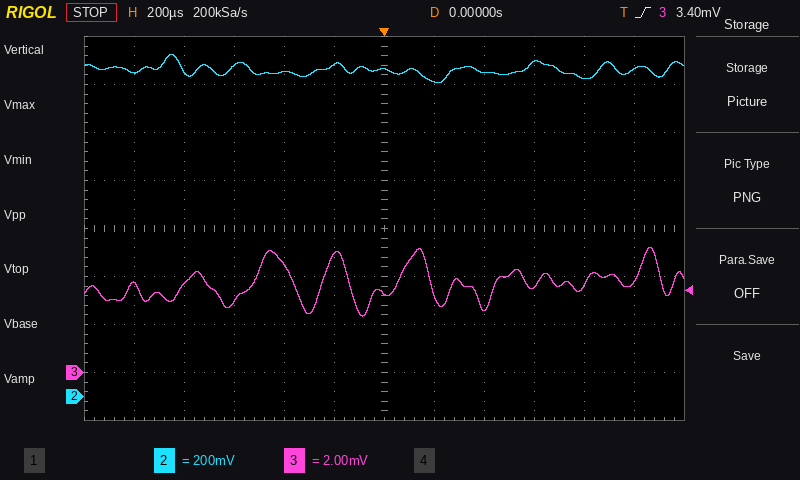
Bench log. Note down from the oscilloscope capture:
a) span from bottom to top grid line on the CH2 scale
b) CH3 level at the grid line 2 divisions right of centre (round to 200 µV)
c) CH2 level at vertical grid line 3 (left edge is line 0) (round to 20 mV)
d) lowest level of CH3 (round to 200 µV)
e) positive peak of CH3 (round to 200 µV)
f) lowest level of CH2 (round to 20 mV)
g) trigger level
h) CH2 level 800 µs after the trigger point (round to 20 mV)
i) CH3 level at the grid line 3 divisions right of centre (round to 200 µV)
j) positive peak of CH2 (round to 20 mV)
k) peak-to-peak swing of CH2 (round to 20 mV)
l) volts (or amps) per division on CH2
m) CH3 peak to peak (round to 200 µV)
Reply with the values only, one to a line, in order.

1.6 V
2.6 mV
1.38 V
2.4 mV
5.2 mV
1.30 V
3.40 mV
1.32 V
3.6 mV
1.42 V
120 mV
200 mV
2.8 mV
